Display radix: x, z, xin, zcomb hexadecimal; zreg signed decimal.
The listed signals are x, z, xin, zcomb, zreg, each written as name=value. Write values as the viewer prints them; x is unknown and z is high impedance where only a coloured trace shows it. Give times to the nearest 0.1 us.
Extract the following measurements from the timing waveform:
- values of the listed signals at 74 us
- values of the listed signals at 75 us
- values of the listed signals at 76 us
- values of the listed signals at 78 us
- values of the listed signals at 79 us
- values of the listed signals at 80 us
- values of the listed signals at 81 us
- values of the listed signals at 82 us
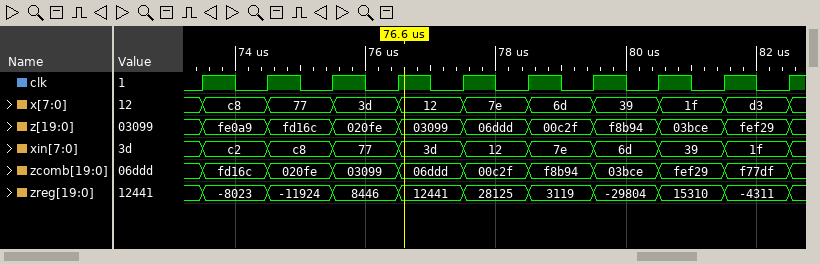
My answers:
x=c8, z=fe0a9, xin=c2, zcomb=fd16c, zreg=-8023
x=77, z=fd16c, xin=c8, zcomb=020fe, zreg=-11924
x=3d, z=020fe, xin=77, zcomb=03099, zreg=8446
x=7e, z=06ddd, xin=12, zcomb=00c2f, zreg=28125
x=6d, z=00c2f, xin=7e, zcomb=f8b94, zreg=3119
x=39, z=f8b94, xin=6d, zcomb=03bce, zreg=-29804
x=1f, z=03bce, xin=39, zcomb=fef29, zreg=15310
x=d3, z=fef29, xin=1f, zcomb=f77df, zreg=-4311
